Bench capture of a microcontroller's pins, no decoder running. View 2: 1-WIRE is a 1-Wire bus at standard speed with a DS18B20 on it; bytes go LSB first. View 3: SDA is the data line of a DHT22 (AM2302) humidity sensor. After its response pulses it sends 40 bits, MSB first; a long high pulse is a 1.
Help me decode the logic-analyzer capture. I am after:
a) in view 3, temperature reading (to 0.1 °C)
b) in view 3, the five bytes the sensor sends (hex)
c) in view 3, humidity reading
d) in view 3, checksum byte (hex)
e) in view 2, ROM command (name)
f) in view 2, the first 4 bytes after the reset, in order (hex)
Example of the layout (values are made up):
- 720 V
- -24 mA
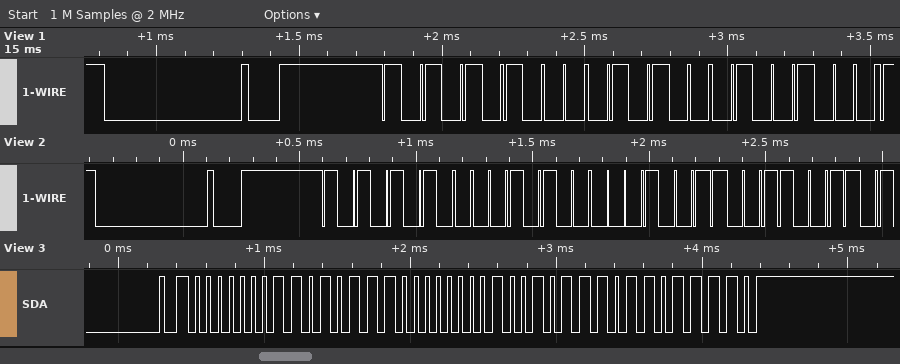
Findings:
- 30.2 °C
- 01 AE 01 2E DE
- 43.0 %
- 0xDE
- Match ROM
- 55 28 C8 CC
